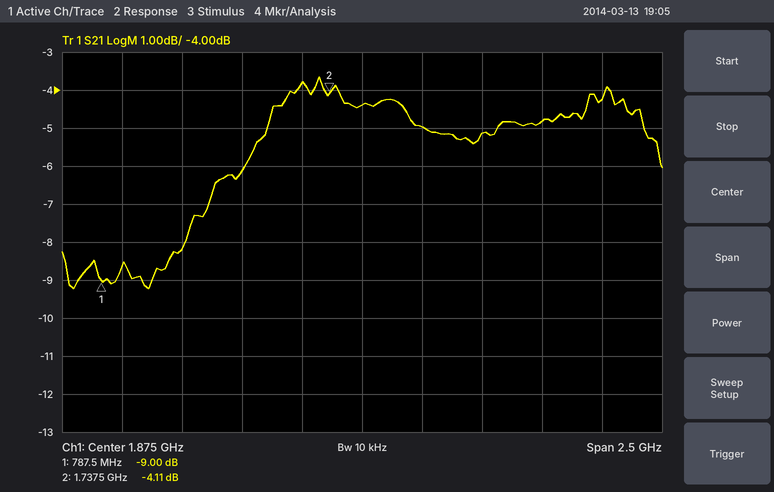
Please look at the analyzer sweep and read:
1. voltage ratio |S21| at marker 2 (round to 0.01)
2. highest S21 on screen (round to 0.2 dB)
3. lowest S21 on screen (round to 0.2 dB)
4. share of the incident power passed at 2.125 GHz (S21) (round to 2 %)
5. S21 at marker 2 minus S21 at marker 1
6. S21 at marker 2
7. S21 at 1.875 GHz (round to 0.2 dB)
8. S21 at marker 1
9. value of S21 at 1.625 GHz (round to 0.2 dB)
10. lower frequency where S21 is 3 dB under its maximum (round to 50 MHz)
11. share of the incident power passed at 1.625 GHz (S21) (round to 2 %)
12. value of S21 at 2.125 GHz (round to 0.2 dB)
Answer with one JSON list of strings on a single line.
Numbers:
["0.62", "-3.6 dB", "-9.2 dB", "32 %", "4.89 dB", "-4.11 dB", "-4.4 dB", "-9.00 dB", "-3.8 dB", "1.25 GHz", "42 %", "-5.0 dB"]
